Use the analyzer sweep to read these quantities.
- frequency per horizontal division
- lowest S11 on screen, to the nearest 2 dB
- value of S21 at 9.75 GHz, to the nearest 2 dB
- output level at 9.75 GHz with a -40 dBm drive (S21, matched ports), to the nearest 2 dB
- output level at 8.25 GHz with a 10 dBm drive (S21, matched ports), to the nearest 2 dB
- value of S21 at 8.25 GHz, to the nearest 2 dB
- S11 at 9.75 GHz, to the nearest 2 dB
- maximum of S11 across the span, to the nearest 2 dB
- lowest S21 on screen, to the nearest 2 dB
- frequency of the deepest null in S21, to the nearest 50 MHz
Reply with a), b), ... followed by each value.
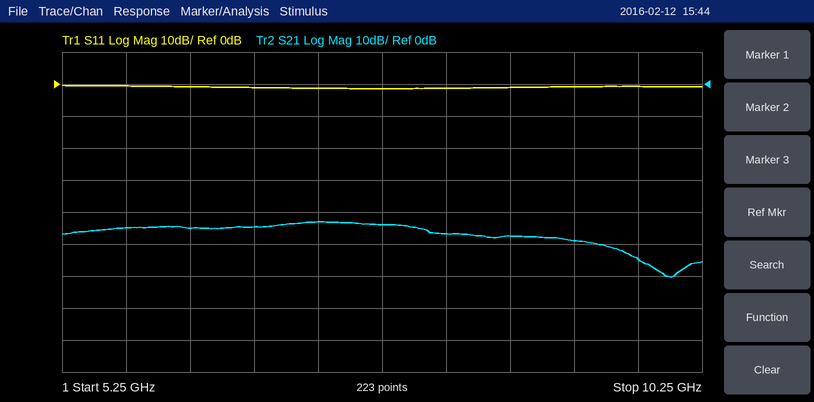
a) 500 MHz
b) -2 dB
c) -54 dB
d) -94 dBm
e) -36 dBm
f) -46 dB
g) 0 dB
h) 0 dB
i) -60 dB
j) 10.00 GHz
